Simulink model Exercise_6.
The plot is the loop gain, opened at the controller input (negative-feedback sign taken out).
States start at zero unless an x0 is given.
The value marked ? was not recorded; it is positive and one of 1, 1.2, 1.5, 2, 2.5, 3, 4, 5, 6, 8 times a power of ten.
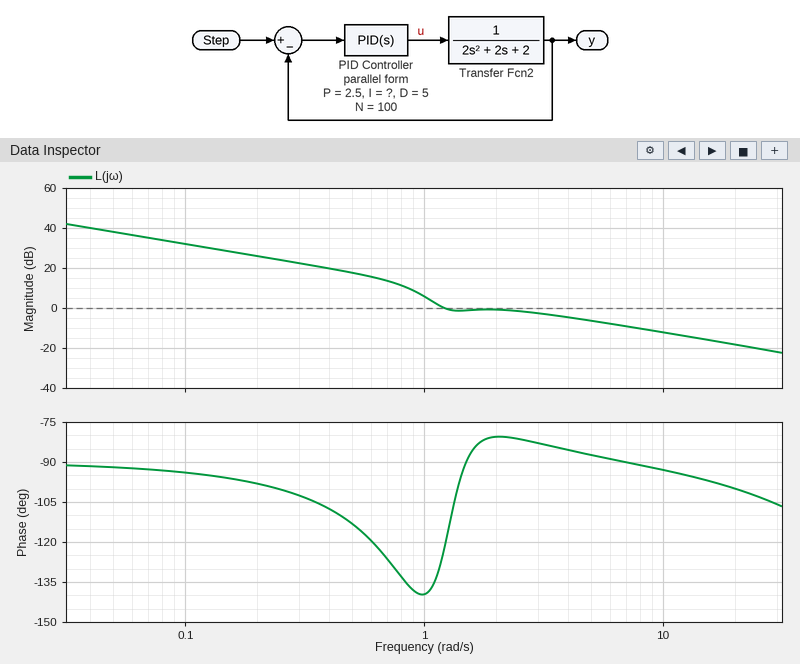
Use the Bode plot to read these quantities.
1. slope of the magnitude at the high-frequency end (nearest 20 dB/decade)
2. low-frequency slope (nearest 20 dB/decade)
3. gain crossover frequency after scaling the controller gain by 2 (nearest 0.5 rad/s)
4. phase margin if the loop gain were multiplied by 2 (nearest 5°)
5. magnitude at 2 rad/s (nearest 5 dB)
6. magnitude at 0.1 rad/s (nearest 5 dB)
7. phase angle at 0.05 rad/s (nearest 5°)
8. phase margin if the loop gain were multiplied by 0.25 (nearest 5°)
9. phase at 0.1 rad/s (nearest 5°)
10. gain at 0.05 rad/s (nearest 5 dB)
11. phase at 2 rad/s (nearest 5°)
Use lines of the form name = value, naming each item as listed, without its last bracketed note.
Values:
slope of the magnitude at the high-frequency end = -20 dB/decade
low-frequency slope = -20 dB/decade
gain crossover frequency after scaling the controller gain by 2 = 5.0 rad/s
phase margin if the loop gain were multiplied by 2 = 95°
magnitude at 2 rad/s = 0 dB
magnitude at 0.1 rad/s = 30 dB
phase angle at 0.05 rad/s = -90°
phase margin if the loop gain were multiplied by 0.25 = 50°
phase at 0.1 rad/s = -95°
gain at 0.05 rad/s = 40 dB
phase at 2 rad/s = -80°
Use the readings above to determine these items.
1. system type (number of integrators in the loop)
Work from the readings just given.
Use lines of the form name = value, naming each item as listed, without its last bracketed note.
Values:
system type = 1
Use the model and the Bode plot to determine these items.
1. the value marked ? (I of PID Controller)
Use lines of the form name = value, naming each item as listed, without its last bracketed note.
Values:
the value marked ? = 8
